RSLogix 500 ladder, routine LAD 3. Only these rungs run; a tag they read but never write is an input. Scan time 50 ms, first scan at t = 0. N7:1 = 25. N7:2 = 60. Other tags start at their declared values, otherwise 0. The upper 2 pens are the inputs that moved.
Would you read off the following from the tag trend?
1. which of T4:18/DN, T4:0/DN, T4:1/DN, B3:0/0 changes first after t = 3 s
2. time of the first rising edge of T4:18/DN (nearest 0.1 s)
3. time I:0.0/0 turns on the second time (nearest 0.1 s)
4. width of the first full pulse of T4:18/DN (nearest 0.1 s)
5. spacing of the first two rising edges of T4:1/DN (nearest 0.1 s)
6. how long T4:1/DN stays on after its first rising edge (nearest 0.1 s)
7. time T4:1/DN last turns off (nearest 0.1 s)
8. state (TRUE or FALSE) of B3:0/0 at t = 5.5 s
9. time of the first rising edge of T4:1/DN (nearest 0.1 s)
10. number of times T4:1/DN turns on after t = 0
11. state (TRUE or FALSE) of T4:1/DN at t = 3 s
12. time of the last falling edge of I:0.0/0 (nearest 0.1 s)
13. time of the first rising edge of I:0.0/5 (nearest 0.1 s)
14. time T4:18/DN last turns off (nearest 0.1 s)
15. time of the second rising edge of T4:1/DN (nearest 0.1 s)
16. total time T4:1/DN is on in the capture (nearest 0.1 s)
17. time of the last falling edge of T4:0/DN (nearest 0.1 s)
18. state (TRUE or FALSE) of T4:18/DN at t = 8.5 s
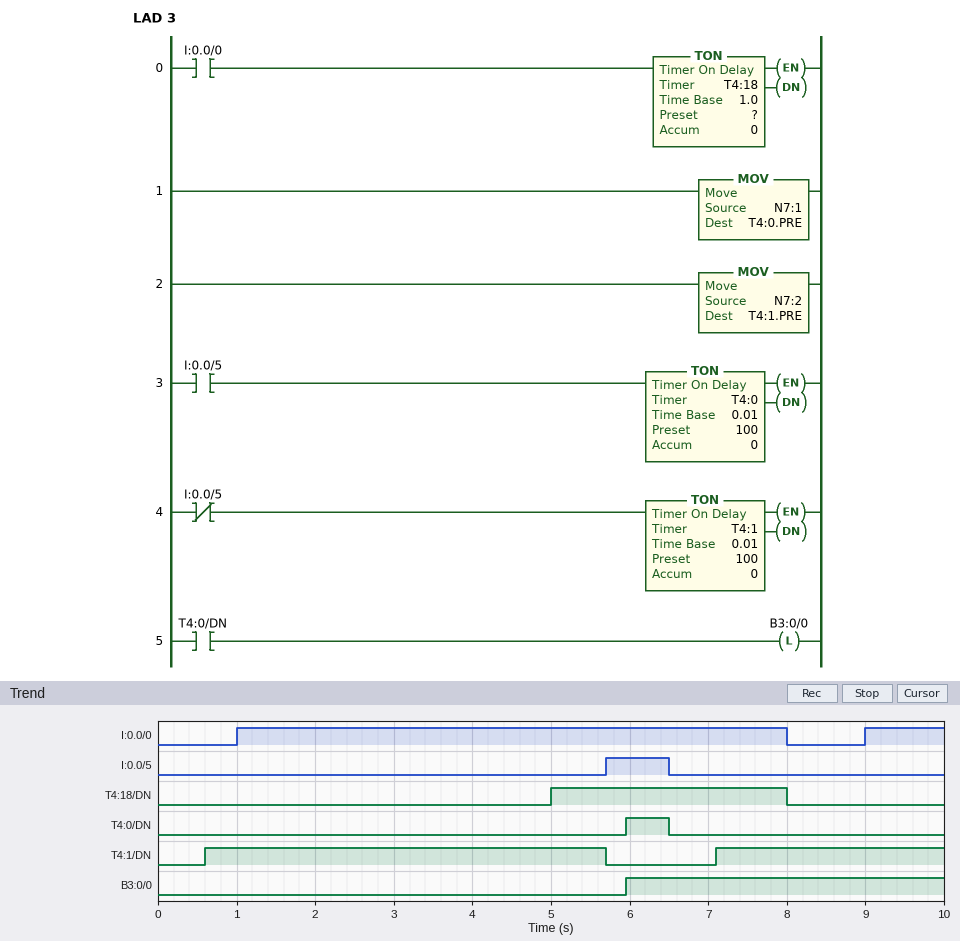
T4:18/DN
5.0 s
9.0 s
3.0 s
6.5 s
5.1 s
5.7 s
FALSE
0.6 s
2
TRUE
8.0 s
5.7 s
8.0 s
7.1 s
8.0 s
6.5 s
FALSE
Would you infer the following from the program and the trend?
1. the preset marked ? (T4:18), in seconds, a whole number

4 s
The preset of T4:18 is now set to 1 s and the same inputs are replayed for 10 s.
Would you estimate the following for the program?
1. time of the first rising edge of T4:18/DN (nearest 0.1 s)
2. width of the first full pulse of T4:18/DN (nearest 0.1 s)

2.0 s
6.0 s
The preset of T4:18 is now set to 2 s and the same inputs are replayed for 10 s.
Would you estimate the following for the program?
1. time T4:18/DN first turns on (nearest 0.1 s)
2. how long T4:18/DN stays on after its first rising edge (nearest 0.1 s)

3.0 s
5.0 s
